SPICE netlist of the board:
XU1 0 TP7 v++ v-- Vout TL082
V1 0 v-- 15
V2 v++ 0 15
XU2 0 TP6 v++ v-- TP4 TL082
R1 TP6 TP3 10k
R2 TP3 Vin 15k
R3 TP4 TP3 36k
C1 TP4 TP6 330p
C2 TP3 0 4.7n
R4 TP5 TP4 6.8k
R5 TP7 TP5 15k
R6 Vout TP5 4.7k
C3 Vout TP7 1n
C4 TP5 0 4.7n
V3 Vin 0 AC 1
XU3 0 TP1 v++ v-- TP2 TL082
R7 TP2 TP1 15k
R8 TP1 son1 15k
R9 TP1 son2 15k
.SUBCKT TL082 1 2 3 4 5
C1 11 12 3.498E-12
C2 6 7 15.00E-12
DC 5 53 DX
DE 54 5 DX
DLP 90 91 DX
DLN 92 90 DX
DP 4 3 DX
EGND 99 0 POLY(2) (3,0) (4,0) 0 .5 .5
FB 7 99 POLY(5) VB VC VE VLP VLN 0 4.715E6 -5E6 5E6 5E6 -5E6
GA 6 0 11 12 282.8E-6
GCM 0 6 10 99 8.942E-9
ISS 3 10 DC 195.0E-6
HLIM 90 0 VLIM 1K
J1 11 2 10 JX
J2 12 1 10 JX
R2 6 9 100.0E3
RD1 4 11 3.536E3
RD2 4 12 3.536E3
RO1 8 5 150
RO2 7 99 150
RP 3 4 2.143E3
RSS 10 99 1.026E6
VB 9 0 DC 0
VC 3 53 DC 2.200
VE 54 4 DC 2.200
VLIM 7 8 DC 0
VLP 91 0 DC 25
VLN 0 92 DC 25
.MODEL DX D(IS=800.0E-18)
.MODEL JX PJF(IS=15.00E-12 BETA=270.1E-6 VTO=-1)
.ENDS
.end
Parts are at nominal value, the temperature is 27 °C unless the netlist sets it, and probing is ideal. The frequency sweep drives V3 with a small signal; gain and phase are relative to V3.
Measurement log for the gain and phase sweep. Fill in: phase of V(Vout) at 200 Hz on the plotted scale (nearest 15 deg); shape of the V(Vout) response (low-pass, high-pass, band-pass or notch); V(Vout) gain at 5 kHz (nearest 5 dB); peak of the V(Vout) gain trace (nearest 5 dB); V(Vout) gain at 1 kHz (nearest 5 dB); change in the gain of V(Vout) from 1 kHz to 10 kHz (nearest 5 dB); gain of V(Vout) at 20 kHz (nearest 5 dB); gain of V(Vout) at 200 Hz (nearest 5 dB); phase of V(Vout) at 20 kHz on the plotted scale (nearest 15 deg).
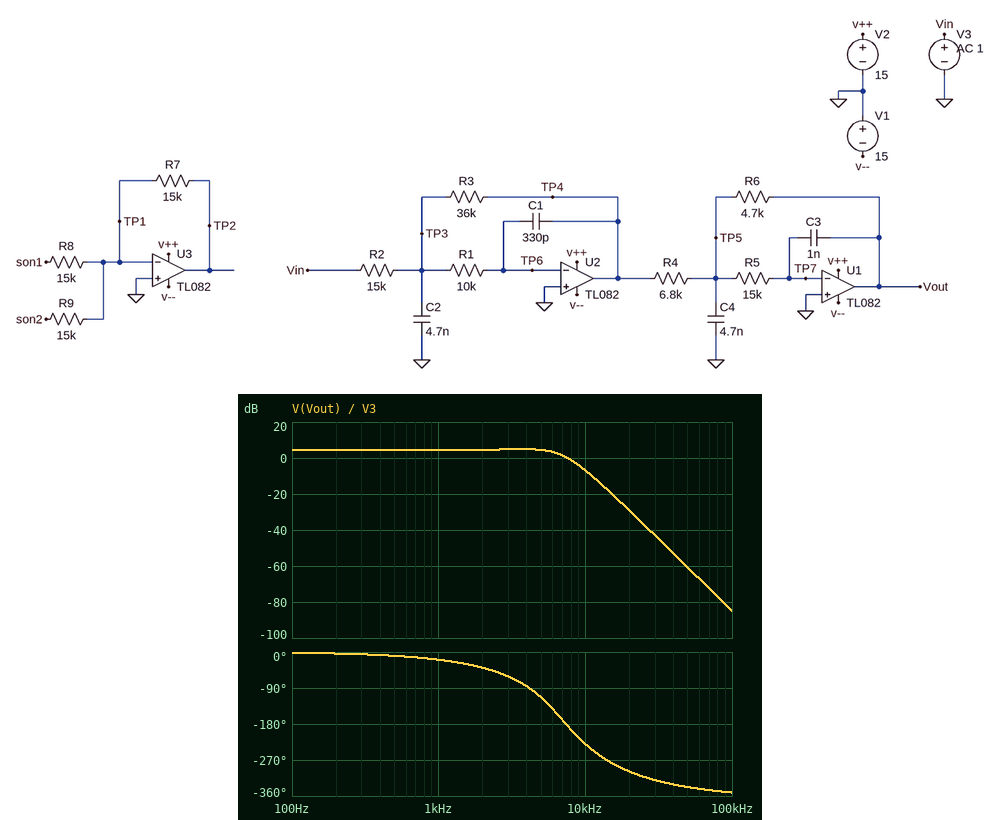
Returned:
0 deg
low-pass
5 dB
5 dB
5 dB
-10 dB
-30 dB
5 dB
-300 deg
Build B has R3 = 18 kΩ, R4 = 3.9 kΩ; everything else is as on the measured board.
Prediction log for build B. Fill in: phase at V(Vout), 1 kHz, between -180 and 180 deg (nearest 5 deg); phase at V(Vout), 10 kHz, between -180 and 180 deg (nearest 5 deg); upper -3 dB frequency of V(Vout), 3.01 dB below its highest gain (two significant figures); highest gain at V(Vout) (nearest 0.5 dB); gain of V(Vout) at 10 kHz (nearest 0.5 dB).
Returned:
-20 deg
165 deg
8.2 kHz
3.0 dB
-3.0 dB
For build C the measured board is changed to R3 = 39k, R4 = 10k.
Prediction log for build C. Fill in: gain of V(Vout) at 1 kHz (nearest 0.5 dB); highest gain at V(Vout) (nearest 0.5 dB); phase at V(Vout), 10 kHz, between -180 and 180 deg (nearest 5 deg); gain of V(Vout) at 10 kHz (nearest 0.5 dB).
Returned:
2.0 dB
2.5 dB
125 deg
-9.5 dB
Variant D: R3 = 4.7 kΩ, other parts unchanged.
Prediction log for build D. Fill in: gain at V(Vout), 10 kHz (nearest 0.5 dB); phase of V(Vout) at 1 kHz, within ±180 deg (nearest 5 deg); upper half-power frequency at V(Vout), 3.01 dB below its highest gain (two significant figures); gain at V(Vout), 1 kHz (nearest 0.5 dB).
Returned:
-17.0 dB
-15 deg
9.0 kHz
-13.5 dB
